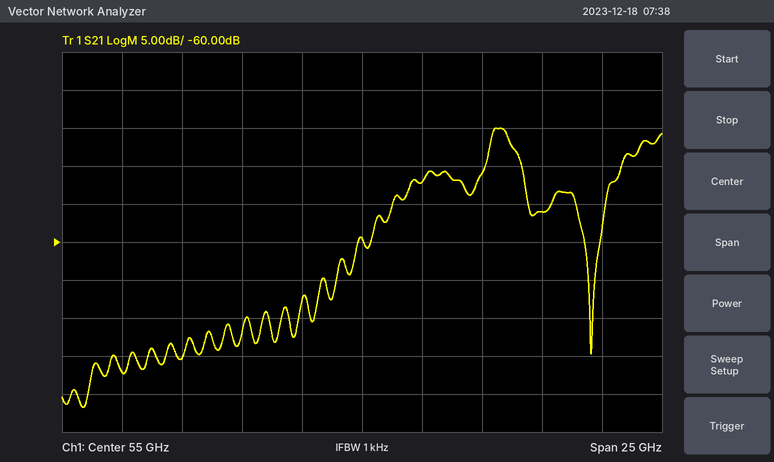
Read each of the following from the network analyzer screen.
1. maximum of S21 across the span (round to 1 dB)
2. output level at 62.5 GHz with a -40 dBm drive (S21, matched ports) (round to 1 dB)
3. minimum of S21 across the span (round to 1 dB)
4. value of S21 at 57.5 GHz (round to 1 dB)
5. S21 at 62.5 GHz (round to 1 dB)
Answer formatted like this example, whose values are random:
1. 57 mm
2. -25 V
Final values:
1. -45 dB
2. -96 dBm
3. -82 dB
4. -52 dB
5. -56 dB
